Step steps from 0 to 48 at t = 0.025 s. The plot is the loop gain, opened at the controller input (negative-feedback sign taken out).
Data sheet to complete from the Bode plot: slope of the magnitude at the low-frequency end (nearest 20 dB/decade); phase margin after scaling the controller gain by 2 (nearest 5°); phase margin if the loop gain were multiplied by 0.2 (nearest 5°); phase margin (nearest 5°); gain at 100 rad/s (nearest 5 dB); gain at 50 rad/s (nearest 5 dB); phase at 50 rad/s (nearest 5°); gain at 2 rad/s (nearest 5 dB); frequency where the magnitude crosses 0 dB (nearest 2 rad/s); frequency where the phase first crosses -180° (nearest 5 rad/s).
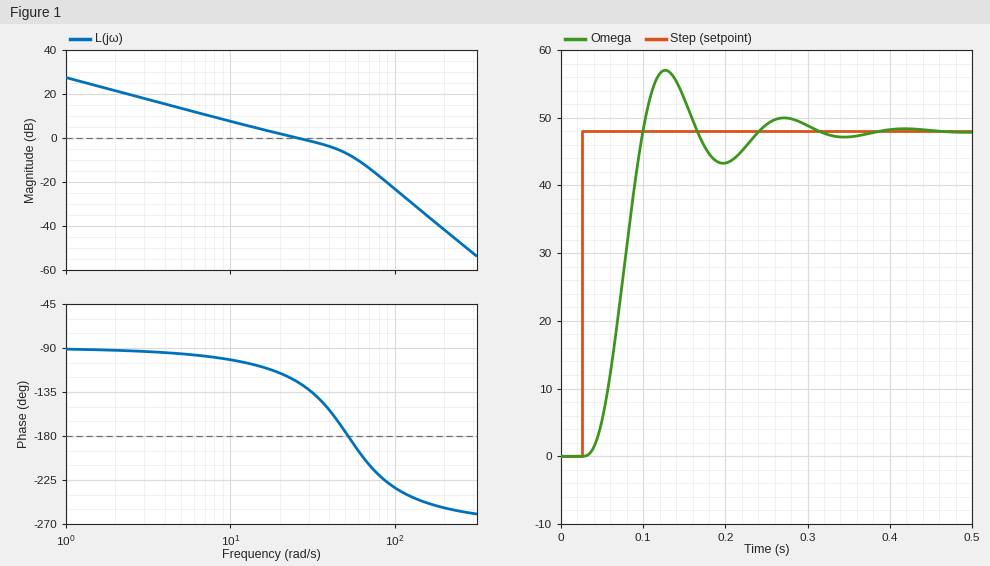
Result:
-20 dB/decade
10°
85°
55°
-25 dB
-5 dB
-175°
20 dB
26 rad/s
50 rad/s
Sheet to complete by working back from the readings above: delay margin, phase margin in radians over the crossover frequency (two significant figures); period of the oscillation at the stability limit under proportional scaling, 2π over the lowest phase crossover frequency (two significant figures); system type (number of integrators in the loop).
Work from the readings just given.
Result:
0.037 s
0.13 s
1
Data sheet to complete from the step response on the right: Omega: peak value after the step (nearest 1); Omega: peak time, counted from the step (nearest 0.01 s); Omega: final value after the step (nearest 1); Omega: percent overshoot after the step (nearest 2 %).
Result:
57
0.10 s
48
18 %
